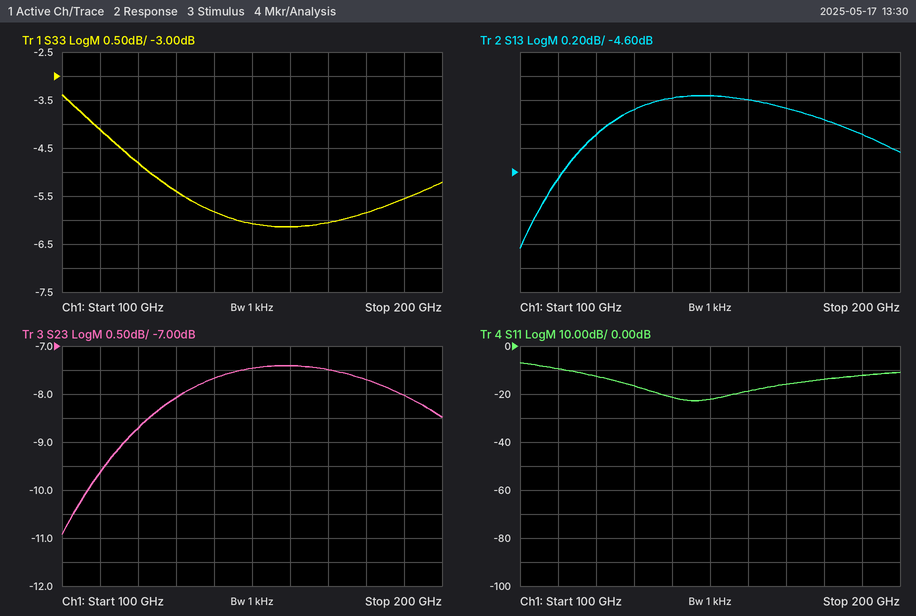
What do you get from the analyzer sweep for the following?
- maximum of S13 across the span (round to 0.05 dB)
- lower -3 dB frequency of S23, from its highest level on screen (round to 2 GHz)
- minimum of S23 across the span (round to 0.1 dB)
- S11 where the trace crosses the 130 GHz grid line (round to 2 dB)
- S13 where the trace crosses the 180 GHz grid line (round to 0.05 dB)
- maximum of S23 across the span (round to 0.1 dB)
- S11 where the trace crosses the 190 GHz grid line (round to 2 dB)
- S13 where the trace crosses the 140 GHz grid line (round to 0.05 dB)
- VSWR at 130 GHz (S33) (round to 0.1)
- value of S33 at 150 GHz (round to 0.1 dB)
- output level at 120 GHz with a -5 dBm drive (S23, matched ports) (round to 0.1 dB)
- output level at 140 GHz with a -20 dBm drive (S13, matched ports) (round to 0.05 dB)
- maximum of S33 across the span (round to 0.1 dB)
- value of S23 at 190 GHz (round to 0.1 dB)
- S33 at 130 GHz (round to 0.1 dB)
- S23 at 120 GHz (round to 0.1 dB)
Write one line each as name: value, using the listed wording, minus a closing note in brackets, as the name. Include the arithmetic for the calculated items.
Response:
maximum of S13 across the span: -3.95 dB
lower -3 dB frequency of S23, from its highest level on screen: 104 GHz
minimum of S23 across the span: -10.9 dB
S11 where the trace crosses the 130 GHz grid line: -16 dB
S13 where the trace crosses the 180 GHz grid line: -4.15 dB
maximum of S23 across the span: -7.4 dB
S11 where the trace crosses the 190 GHz grid line: -12 dB
S13 where the trace crosses the 140 GHz grid line: -4.00 dB
VSWR at 130 GHz (S33): |Γ| = 10^(-5.4/20) = 0.5370; VSWR = (1 + 0.5370)/(1 − 0.5370) ≈ 3.3
value of S33 at 150 GHz: -6.1 dB
output level at 120 GHz with a -5 dBm drive (S23, matched ports): -5 dBm + (-8.7 dB) = -13.7 dBm
output level at 140 GHz with a -20 dBm drive (S13, matched ports): -20 dBm + (-4.00 dB) = -24.00 dBm
maximum of S33 across the span: -3.4 dB
value of S23 at 190 GHz: -8.0 dB
S33 at 130 GHz: -5.4 dB
S23 at 120 GHz: -8.7 dB
